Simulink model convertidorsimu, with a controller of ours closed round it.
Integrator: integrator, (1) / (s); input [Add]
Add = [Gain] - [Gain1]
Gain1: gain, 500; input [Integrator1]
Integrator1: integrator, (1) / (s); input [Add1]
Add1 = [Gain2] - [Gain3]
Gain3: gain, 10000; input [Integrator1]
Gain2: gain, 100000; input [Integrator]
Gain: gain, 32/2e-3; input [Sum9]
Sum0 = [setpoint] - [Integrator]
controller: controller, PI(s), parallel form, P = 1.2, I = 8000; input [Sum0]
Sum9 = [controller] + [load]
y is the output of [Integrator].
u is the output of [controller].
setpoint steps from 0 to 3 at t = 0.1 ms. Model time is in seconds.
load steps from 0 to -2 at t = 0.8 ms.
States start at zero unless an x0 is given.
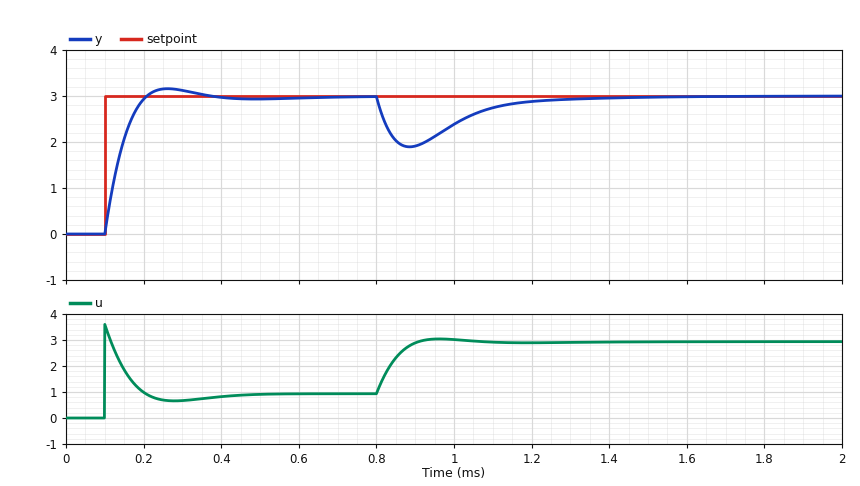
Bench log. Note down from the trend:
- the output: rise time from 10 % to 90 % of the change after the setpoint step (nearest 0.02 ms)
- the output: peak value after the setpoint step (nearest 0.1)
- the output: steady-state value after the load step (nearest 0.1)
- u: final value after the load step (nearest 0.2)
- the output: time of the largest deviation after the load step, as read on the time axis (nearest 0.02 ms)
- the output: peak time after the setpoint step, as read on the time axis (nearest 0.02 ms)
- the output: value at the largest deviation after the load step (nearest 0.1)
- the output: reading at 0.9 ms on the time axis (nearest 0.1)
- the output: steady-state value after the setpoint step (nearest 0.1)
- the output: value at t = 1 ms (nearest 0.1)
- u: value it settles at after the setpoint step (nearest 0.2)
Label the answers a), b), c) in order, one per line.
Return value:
a) 0.08 ms
b) 3.2
c) 3.0
d) 3.0
e) 0.88 ms
f) 0.26 ms
g) 1.9
h) 1.9
i) 3.0
j) 2.4
k) 1.0
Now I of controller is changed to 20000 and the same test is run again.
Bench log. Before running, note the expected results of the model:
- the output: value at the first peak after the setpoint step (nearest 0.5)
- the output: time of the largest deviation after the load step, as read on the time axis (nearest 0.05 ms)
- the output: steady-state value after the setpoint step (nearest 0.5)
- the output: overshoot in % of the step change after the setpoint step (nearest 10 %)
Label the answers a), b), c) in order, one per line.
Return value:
a) 3.5
b) 0.85 ms
c) 3.0
d) 20 %
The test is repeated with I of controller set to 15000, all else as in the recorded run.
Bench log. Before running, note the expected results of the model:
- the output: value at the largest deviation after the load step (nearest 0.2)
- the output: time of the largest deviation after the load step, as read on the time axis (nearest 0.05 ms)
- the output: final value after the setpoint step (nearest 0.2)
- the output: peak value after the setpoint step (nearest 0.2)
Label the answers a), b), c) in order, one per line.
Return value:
a) 2.0
b) 0.85 ms
c) 3.0
d) 3.4
